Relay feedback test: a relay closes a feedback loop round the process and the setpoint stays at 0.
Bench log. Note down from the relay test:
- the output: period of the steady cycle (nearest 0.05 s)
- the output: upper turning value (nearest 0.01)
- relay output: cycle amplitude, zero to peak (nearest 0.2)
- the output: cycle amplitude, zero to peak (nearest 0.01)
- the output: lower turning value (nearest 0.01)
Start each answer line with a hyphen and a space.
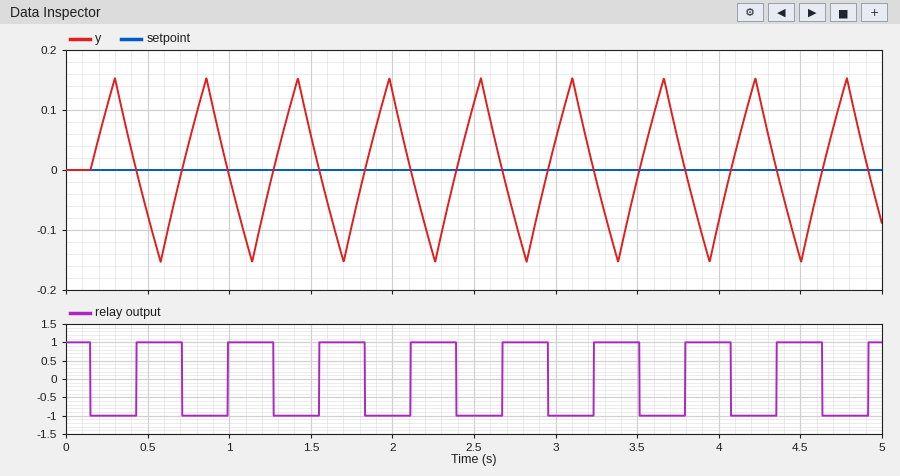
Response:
- 0.55 s
- 0.15
- 1.0
- 0.15
- -0.15
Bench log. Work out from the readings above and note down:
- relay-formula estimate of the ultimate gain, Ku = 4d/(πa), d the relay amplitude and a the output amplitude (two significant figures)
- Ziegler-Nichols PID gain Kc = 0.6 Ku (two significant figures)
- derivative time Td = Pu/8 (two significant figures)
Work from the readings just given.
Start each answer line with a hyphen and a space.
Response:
- 8.5
- 5.1
- 0.069 s
